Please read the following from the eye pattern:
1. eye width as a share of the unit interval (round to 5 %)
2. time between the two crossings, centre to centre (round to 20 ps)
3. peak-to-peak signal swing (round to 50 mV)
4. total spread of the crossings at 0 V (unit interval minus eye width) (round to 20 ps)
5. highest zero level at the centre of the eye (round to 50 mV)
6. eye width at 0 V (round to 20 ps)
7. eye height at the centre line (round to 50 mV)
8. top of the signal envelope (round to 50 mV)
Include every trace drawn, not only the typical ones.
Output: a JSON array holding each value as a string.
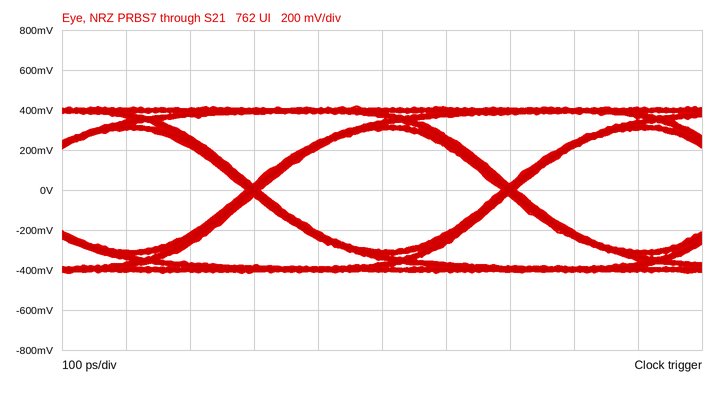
["95 %", "400 ps", "850 mV", "20 ps", "-300 mV", "380 ps", "600 mV", "400 mV"]
